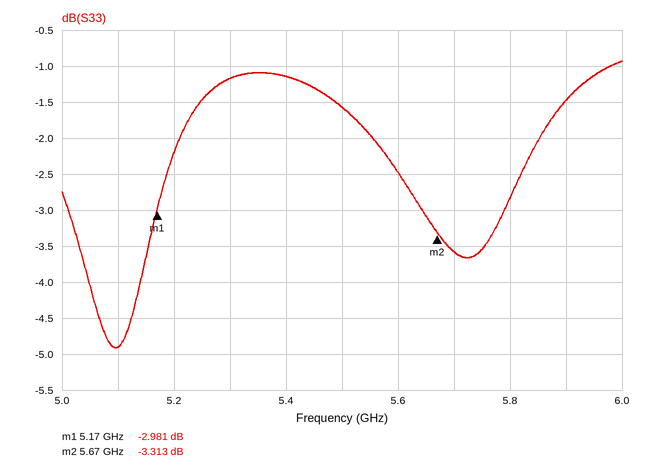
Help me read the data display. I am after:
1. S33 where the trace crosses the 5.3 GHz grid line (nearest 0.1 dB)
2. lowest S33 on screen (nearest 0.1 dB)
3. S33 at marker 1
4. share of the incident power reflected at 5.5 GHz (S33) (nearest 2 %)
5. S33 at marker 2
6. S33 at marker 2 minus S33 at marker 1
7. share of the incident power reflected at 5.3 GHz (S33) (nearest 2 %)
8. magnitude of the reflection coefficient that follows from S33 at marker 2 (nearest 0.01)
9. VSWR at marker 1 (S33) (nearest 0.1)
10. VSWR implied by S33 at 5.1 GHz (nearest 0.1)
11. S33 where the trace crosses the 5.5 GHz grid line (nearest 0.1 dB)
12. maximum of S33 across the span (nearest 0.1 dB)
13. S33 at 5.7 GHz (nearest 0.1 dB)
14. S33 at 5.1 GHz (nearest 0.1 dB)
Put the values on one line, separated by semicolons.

-1.2 dB; -4.9 dB; -2.981 dB; 70 %; -3.313 dB; -0.332 dB; 76 %; 0.68; 5.9; 3.6; -1.6 dB; -0.9 dB; -3.6 dB; -4.9 dB
